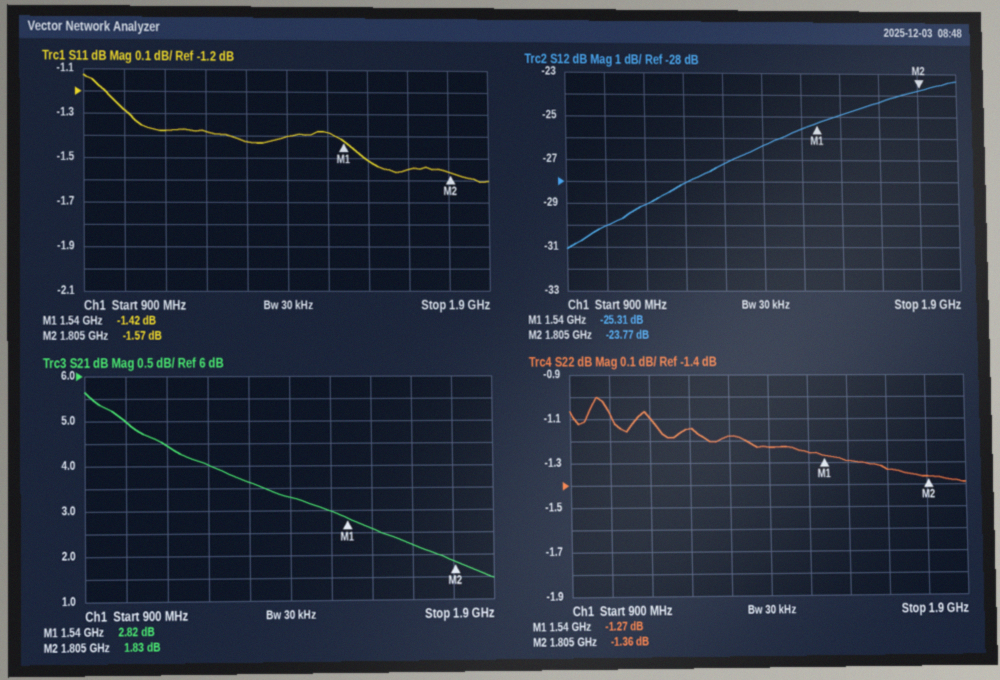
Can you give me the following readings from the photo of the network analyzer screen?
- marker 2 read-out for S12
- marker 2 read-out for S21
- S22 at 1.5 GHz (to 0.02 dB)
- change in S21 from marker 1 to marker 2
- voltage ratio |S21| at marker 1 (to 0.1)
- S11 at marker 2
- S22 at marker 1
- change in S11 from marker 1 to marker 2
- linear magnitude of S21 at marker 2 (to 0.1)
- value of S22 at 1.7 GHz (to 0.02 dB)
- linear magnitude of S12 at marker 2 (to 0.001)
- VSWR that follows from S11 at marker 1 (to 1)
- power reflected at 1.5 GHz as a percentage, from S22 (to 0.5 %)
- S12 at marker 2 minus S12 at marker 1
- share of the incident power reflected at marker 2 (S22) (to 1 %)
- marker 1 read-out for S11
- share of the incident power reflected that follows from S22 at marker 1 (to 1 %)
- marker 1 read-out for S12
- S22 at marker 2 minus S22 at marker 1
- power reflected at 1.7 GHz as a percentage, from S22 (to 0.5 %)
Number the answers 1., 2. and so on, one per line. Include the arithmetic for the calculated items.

1. -23.77 dB
2. 1.83 dB
3. -1.26 dB
4. 1.83 − (2.82) = -0.99 dB
5. 10^(2.82/20) ≈ 1.4
6. -1.57 dB
7. -1.27 dB
8. -1.57 − (-1.42) = -0.15 dB
9. 10^(1.83/20) ≈ 1.2
10. -1.34 dB
11. 10^(-23.77/20) ≈ 0.065
12. (1 + 0.8492)/(1 − 0.8492) ≈ 12
13. 10^(-1.26/10) ≈ 74.8 %, so 75.0 % to the nearest 0.5 %
14. -23.77 − (-25.31) = 1.54 dB
15. 10^(-1.36/10) ≈ 73 %
16. -1.42 dB
17. 10^(-1.27/10) ≈ 75 %
18. -25.31 dB
19. -1.36 − (-1.27) = -0.09 dB
20. 10^(-1.34/10) ≈ 73.5 %
